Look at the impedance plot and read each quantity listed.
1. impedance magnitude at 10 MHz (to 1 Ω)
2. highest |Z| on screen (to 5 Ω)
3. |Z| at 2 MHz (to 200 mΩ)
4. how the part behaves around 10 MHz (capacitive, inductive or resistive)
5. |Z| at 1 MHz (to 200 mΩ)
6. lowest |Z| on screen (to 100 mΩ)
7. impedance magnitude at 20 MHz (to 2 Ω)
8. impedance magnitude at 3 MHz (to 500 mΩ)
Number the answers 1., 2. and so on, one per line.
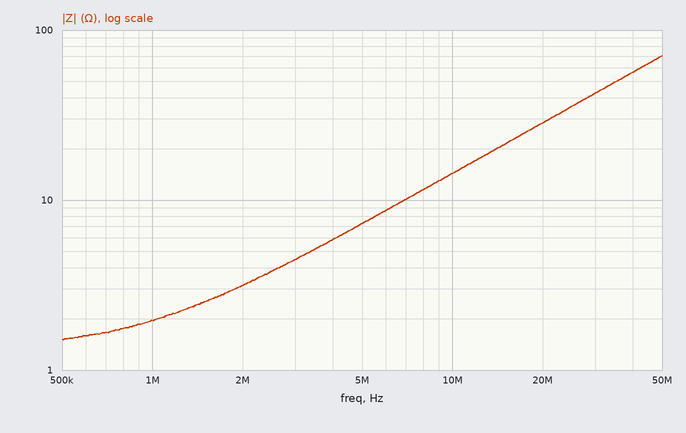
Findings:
1. 14 Ω
2. 70 Ω
3. 3.2 Ω
4. inductive
5. 2.0 Ω
6. 1.5 Ω
7. 28 Ω
8. 4.5 Ω
